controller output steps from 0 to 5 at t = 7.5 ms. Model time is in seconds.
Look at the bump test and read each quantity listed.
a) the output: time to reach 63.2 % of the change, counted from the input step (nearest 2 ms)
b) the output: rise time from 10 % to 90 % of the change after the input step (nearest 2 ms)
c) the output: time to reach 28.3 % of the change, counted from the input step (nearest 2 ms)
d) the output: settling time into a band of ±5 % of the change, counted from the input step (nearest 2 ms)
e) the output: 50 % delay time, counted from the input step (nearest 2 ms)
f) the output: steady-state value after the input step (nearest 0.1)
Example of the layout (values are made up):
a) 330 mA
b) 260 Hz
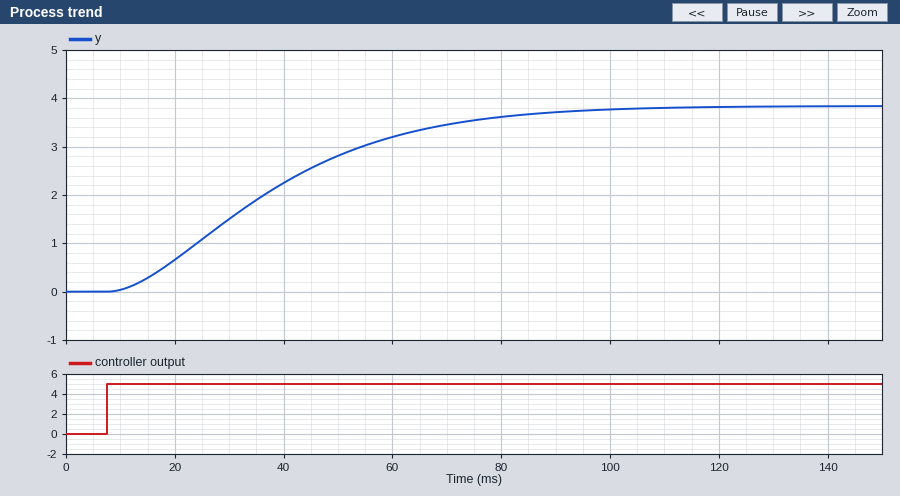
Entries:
a) 36 ms
b) 54 ms
c) 18 ms
d) 76 ms
e) 28 ms
f) 3.8
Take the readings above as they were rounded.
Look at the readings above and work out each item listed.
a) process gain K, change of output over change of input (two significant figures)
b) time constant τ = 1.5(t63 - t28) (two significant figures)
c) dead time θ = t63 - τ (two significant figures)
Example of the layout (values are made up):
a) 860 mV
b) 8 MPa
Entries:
a) 0.76
b) 27 ms
c) 9.0 ms
